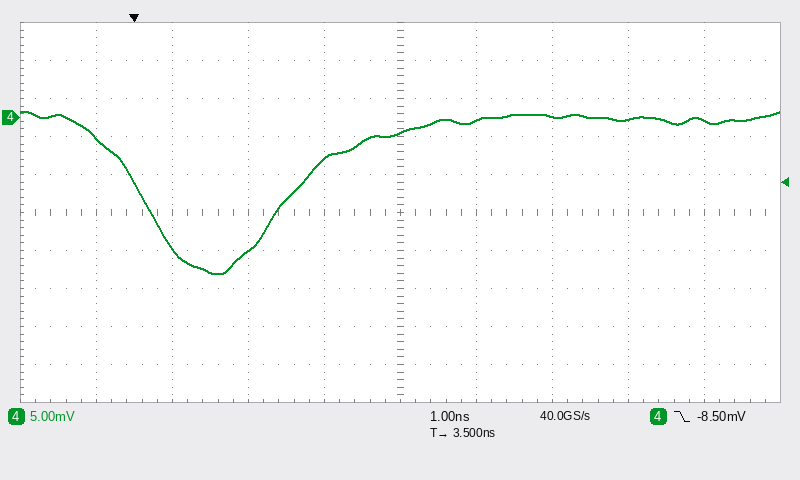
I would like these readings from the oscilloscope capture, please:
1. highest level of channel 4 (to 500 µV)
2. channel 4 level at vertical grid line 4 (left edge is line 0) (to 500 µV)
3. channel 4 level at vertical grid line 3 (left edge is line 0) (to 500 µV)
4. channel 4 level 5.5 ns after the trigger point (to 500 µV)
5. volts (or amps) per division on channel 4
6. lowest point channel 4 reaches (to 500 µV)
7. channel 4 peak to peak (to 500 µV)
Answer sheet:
1.0 mV
-5.5 mV
-17.5 mV
0.0 mV
5 mV
-20.5 mV
21.5 mV
